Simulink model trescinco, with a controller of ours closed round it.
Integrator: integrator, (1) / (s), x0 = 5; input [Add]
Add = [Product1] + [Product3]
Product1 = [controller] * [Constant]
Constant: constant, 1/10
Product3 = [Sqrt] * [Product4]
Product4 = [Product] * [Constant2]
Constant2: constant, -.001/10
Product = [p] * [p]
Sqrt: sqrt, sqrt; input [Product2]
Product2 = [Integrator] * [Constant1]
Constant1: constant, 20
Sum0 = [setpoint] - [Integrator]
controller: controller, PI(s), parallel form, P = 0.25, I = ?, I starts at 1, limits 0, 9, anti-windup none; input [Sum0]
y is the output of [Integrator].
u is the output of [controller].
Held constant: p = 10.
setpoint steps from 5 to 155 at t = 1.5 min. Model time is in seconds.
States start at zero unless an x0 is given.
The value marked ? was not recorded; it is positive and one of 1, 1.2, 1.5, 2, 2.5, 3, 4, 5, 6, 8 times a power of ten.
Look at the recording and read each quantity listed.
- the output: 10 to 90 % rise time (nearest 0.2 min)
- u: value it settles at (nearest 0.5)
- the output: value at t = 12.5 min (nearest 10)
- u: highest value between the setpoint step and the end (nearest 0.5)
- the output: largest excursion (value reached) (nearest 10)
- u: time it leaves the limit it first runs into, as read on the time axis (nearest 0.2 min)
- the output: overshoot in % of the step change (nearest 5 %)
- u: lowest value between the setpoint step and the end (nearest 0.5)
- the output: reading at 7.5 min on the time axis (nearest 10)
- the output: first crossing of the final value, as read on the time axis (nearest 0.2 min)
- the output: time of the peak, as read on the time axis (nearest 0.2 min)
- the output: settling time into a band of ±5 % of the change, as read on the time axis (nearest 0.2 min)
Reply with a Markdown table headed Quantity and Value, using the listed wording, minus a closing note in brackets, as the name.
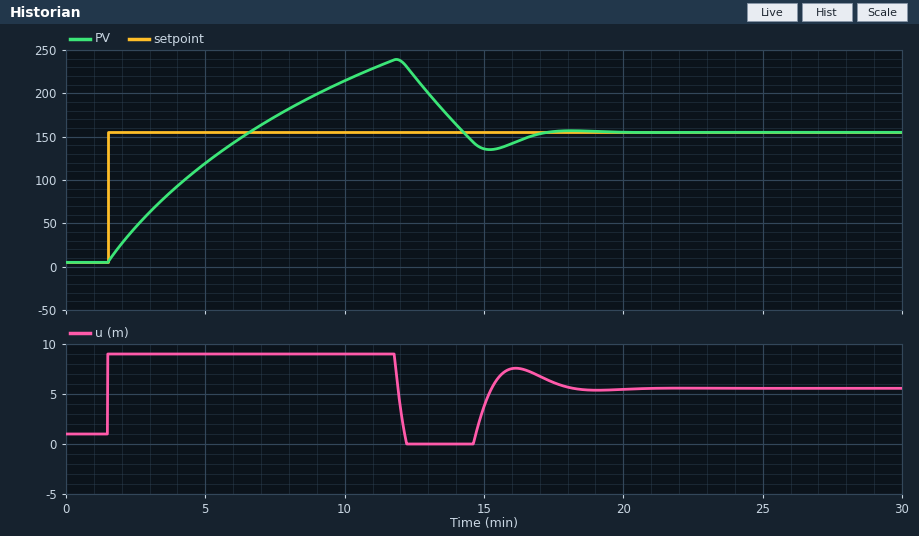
| Quantity | Value |
|---|---|
| the output: 10 to 90 % rise time | 4.0 min |
| u: value it settles at | 5.5 |
| the output: value at t = 12.5 min | 220 |
| u: highest value between the setpoint step and the end | 9.0 |
| the output: largest excursion (value reached) | 240 |
| u: time it leaves the limit it first runs into, as read on the time axis | 11.8 min |
| the output: overshoot in % of the step change | 55 % |
| u: lowest value between the setpoint step and the end | 0.0 |
| the output: reading at 7.5 min on the time axis | 170 |
| the output: first crossing of the final value, as read on the time axis | 6.6 min |
| the output: time of the peak, as read on the time axis | 11.8 min |
| the output: settling time into a band of ±5 % of the change, as read on the time axis | 16.4 min |
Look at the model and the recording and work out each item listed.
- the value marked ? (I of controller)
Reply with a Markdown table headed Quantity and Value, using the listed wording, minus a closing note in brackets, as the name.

| Quantity | Value |
|---|---|
| the value marked ? | 0.005 |
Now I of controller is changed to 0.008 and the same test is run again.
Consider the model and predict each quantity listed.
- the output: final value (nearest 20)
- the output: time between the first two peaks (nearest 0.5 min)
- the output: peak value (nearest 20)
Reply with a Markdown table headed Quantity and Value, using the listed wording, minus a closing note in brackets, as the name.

| Quantity | Value |
|---|---|
| the output: final value | 160 |
| the output: time between the first two peaks | 7.0 min |
| the output: peak value | 240 |
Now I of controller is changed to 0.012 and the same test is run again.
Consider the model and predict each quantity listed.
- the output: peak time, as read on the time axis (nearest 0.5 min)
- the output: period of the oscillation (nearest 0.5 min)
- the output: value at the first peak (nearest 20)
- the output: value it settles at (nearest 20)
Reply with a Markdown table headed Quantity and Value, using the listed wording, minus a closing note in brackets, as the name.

| Quantity | Value |
|---|---|
| the output: peak time, as read on the time axis | 12.5 min |
| the output: period of the oscillation | 8.5 min |
| the output: value at the first peak | 240 |
| the output: value it settles at | 160 |
